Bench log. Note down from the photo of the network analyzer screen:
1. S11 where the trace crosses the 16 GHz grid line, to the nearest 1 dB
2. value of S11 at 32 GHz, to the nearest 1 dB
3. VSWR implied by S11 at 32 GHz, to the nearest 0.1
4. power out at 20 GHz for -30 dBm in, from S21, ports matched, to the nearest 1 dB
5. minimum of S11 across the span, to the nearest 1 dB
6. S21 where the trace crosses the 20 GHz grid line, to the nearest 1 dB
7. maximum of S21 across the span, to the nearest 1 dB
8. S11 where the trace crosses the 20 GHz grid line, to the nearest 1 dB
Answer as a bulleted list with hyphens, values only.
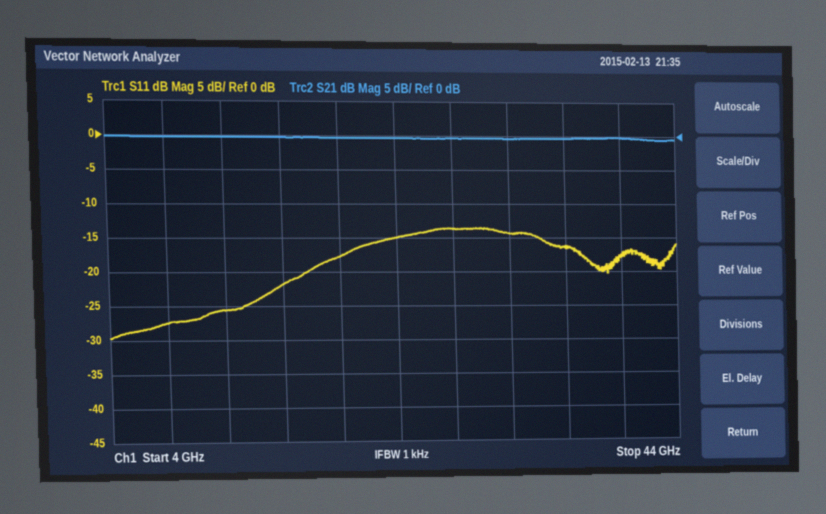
- -22 dB
- -14 dB
- 1.5
- -30 dBm
- -30 dB
- 0 dB
- 0 dB
- -18 dB
